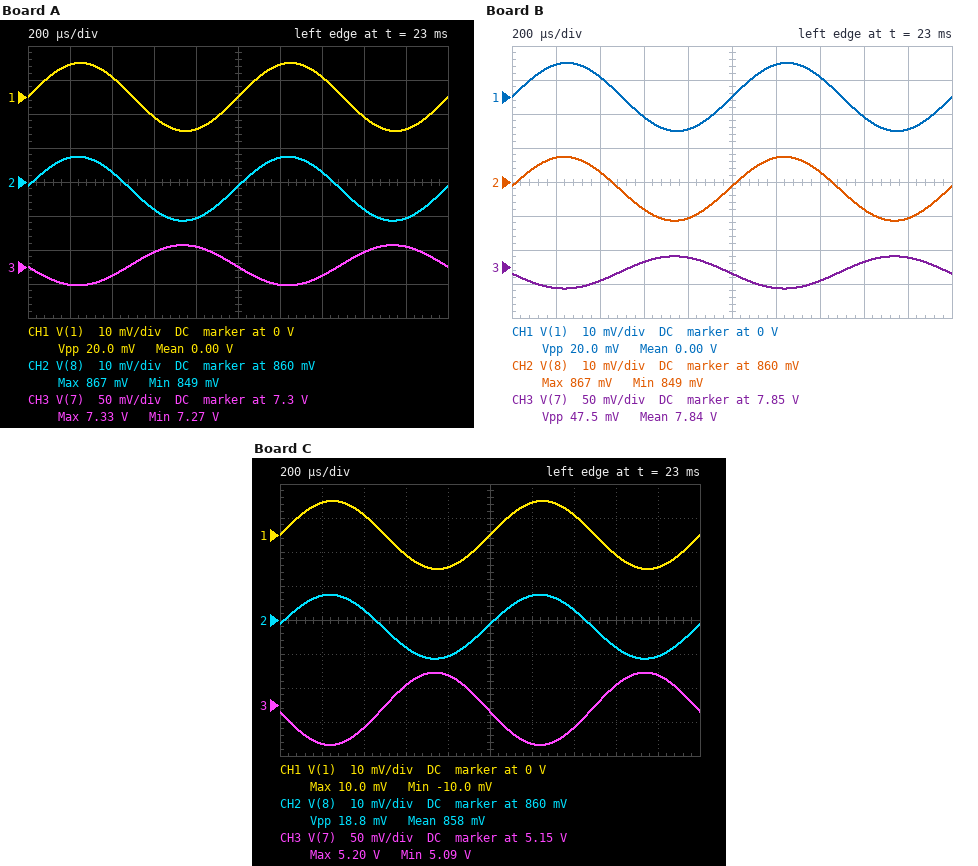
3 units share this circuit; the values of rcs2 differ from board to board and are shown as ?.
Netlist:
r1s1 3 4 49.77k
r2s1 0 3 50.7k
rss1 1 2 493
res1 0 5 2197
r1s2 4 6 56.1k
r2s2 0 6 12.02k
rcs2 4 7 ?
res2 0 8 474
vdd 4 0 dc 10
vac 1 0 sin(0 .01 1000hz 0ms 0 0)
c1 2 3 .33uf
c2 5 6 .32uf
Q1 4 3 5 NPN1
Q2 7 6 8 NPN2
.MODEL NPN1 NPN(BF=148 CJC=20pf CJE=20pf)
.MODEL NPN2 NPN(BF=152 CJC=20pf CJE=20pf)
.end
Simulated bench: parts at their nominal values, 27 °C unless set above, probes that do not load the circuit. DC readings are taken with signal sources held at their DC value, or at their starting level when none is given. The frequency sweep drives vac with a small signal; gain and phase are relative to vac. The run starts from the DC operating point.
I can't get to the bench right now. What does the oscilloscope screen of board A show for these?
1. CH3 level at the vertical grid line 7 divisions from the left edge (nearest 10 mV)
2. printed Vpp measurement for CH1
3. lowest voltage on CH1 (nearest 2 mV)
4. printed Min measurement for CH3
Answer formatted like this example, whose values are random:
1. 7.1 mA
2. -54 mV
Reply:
1. 7.29 V
2. 20.0 mV
3. -10 mV
4. 7.27 V
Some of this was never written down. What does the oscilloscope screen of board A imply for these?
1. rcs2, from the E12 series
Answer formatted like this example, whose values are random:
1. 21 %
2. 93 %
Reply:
1. 1.5 kΩ
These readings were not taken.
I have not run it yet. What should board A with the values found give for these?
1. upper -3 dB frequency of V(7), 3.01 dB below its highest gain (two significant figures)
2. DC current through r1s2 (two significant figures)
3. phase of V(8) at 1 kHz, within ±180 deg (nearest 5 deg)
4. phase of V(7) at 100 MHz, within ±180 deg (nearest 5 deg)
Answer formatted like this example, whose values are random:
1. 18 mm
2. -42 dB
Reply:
1. 11 MHz
2. 150 µA
3. 5 deg
4. -50 deg
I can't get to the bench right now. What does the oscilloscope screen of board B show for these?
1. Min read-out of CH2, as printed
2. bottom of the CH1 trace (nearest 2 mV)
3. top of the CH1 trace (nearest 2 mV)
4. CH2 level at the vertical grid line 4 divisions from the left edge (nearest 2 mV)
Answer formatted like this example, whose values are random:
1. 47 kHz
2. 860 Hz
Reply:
1. 849 mV
2. -10 mV
3. 10 mV
4. 850 mV
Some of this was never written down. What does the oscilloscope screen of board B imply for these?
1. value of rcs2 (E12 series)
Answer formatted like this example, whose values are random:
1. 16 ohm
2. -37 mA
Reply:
1. 1.2 kΩ
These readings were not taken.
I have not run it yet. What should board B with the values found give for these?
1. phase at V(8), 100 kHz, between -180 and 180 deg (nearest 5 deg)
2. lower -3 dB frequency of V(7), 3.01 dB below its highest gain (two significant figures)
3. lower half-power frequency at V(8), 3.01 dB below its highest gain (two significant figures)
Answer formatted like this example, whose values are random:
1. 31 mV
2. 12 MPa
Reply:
1. 0 deg
2. 63 Hz
3. 63 Hz
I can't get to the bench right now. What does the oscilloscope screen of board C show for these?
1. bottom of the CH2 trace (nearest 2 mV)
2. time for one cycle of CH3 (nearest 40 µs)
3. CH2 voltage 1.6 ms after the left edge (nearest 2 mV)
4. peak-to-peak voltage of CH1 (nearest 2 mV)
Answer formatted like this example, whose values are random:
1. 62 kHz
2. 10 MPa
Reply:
1. 848 mV
2. 1.00 ms
3. 852 mV
4. 20 mV
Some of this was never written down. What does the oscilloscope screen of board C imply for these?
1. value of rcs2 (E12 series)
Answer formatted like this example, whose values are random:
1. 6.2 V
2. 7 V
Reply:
1. 2.7 kΩ
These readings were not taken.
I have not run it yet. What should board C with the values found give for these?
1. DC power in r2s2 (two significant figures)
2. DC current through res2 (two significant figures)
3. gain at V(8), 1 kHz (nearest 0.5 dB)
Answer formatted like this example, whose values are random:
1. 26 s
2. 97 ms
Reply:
1. 230 µW
2. 1.8 mA
3. -0.5 dB
